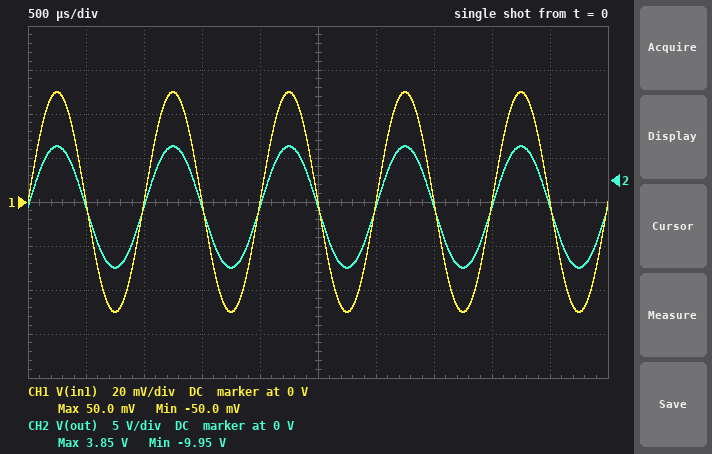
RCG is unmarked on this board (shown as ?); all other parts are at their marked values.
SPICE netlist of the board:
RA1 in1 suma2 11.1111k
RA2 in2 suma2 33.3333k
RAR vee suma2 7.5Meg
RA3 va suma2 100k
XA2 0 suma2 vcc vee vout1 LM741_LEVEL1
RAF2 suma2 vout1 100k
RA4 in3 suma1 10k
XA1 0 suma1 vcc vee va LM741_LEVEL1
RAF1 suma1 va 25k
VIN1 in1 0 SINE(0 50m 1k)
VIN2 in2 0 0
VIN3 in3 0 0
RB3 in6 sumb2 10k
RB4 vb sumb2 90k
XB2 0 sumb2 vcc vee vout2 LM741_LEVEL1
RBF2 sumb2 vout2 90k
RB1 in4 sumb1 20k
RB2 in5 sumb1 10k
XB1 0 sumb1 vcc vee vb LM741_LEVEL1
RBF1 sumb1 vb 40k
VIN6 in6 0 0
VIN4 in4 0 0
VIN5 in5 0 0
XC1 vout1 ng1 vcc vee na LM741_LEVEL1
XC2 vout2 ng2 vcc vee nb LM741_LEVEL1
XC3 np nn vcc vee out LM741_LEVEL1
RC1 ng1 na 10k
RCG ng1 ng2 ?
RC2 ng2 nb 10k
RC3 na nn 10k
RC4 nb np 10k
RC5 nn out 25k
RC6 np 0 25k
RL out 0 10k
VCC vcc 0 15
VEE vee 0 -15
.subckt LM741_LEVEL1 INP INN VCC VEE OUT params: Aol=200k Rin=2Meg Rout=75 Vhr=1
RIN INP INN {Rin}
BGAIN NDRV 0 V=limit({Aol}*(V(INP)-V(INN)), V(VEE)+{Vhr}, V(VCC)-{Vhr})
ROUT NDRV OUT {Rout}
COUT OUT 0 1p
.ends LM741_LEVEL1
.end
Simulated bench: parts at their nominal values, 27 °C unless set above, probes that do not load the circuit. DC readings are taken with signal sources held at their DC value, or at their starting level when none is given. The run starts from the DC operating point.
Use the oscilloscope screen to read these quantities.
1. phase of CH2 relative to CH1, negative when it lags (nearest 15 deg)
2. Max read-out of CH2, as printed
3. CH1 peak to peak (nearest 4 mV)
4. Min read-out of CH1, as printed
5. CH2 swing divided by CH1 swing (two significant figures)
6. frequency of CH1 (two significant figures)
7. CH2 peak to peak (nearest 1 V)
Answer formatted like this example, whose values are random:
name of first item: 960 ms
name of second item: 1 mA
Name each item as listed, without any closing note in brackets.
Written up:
phase of CH2 relative to CH1, negative when it lags: 0 deg
Max read-out of CH2, as printed: 3.85 V
CH1 peak to peak: 100 mV
Min read-out of CH1, as printed: -50.0 mV
CH2 swing divided by CH1 swing: 140
frequency of CH1: 1.0 kHz
CH2 peak to peak: 14 V
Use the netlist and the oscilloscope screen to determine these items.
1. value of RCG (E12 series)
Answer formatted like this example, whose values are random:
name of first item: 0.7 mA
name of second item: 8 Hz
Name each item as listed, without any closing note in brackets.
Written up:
value of RCG: 3.9 kΩ
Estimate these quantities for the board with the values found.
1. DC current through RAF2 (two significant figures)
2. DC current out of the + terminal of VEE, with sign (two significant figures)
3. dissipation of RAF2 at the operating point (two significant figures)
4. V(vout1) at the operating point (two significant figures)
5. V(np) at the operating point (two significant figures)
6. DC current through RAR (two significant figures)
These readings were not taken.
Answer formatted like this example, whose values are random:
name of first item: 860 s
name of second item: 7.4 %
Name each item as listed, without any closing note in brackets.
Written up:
DC current through RAF2: 2.0 µA
DC current out of the + terminal of VEE, with sign: -2.0 µA
dissipation of RAF2 at the operating point: 400 nW
V(vout1) at the operating point: 200 mV
V(np) at the operating point: -370 mV
DC current through RAR: 2.0 µA
